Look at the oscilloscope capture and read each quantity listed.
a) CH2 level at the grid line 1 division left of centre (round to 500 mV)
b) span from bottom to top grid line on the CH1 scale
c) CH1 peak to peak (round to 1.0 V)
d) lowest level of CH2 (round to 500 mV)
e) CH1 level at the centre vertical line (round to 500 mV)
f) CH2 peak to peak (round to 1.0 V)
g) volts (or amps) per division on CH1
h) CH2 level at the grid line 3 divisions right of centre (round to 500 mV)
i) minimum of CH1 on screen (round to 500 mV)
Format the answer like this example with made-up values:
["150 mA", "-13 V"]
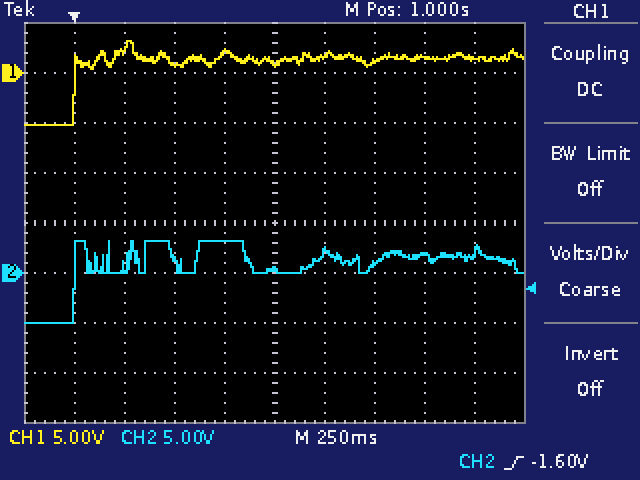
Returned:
["3.0 V", "40 V", "8.0 V", "-5.0 V", "1.0 V", "8.0 V", "5 V", "2.0 V", "-5.0 V"]
